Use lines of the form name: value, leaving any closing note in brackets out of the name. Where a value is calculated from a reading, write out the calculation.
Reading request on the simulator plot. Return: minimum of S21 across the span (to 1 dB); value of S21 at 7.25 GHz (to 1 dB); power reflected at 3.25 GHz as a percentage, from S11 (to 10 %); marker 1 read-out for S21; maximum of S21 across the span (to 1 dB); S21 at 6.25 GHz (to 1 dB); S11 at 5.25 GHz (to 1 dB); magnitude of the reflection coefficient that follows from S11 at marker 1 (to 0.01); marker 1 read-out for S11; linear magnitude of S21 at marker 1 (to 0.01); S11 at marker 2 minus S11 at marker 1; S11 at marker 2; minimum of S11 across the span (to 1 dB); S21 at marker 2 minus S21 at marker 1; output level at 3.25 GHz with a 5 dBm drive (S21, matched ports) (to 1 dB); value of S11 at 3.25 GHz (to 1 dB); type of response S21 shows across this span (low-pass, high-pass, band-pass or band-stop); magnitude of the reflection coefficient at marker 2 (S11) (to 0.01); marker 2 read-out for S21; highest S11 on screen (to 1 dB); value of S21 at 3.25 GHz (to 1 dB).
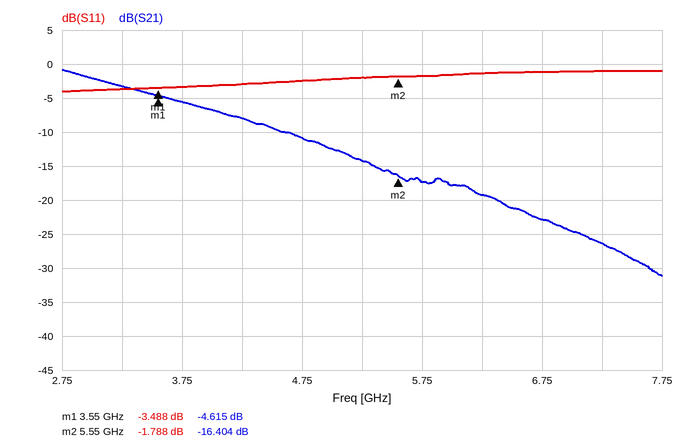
minimum of S21 across the span: -31 dB
value of S21 at 7.25 GHz: -26 dB
power reflected at 3.25 GHz as a percentage, from S11: 10^(-4/10) ≈ 40 %
marker 1 read-out for S21: -4.615 dB
maximum of S21 across the span: -1 dB
S21 at 6.25 GHz: -19 dB
S11 at 5.25 GHz: -2 dB
magnitude of the reflection coefficient that follows from S11 at marker 1: 10^(-3.488/20) ≈ 0.67
marker 1 read-out for S11: -3.488 dB
linear magnitude of S21 at marker 1: 10^(-4.615/20) ≈ 0.59
S11 at marker 2 minus S11 at marker 1: -1.788 − (-3.488) = 1.700 dB
S11 at marker 2: -1.788 dB
minimum of S11 across the span: -4 dB
S21 at marker 2 minus S21 at marker 1: -16.404 − (-4.615) = -11.789 dB
output level at 3.25 GHz with a 5 dBm drive (S21, matched ports): 5 dBm + (-3 dB) = 2 dBm
value of S11 at 3.25 GHz: -4 dB
type of response S21 shows across this span: low-pass
magnitude of the reflection coefficient at marker 2 (S11): 10^(-1.788/20) ≈ 0.81
marker 2 read-out for S21: -16.404 dB
highest S11 on screen: -1 dB
value of S21 at 3.25 GHz: -3 dB
